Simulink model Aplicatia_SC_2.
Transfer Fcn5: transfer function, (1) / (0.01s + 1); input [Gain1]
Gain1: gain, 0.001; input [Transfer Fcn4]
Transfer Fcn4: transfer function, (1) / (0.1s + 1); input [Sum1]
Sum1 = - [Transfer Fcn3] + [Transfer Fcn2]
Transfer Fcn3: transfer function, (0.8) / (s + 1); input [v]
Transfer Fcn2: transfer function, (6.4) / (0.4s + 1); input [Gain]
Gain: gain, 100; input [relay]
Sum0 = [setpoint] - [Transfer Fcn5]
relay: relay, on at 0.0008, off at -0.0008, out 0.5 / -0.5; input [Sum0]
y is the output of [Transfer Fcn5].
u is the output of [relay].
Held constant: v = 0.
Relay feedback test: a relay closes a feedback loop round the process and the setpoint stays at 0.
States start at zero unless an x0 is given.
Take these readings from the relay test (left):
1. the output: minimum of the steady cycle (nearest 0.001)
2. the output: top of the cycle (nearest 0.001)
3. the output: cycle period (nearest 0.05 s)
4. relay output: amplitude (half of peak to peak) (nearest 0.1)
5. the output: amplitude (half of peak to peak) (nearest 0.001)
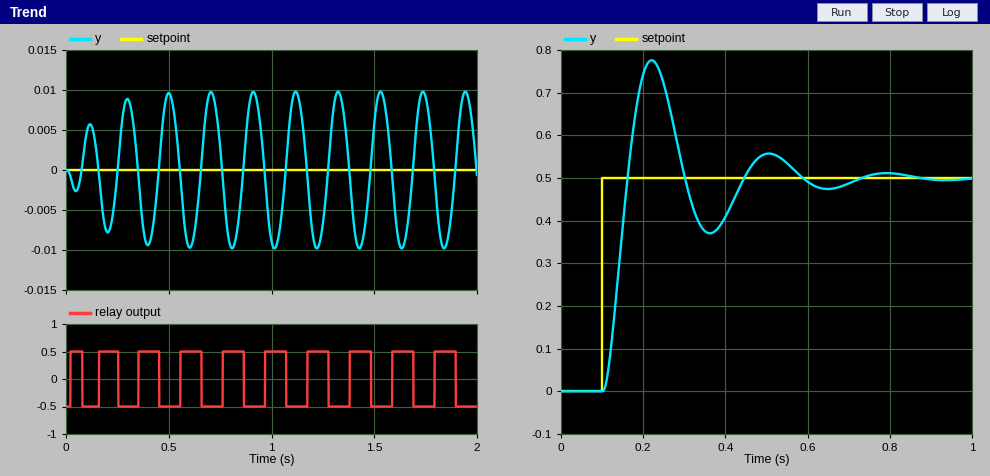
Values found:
-0.010
0.010
0.20 s
0.5
0.010
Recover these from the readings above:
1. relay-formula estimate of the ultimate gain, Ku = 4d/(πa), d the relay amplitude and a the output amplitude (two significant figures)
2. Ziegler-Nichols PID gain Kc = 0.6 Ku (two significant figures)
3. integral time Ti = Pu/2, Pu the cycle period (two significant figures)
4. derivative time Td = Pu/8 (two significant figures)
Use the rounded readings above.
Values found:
64
38
0.10 s
0.025 s
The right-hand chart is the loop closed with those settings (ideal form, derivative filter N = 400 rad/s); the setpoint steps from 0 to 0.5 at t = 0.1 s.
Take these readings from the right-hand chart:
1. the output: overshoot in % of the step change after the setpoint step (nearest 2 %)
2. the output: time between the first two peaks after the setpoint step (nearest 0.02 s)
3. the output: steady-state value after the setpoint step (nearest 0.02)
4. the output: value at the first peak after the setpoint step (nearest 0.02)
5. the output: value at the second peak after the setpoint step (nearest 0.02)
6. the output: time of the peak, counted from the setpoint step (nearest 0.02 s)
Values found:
56 %
0.28 s
0.50
0.78
0.56
0.12 s
